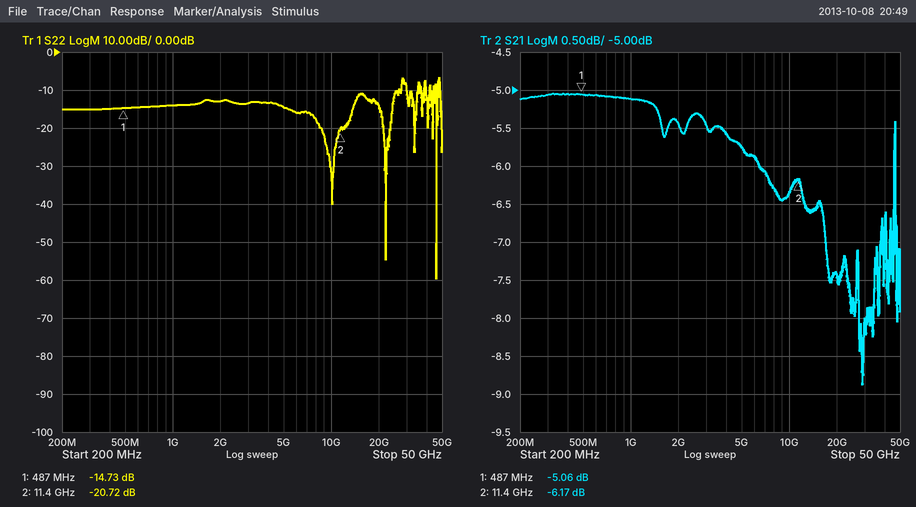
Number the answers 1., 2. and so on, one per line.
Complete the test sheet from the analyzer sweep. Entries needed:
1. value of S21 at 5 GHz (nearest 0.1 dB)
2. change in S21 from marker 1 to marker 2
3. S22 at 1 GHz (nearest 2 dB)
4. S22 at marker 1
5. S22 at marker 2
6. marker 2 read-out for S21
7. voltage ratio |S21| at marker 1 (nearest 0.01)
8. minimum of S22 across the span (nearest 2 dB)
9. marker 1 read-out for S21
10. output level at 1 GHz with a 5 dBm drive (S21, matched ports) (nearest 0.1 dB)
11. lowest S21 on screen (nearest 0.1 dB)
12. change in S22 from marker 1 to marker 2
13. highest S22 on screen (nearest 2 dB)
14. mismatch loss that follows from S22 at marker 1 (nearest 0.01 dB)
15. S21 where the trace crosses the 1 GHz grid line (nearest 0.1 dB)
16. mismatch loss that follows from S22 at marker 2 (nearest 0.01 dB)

1. -5.8 dB
2. -1.11 dB
3. -14 dB
4. -14.73 dB
5. -20.72 dB
6. -6.17 dB
7. 0.56
8. -60 dB
9. -5.06 dB
10. -0.1 dBm
11. -8.9 dB
12. -5.99 dB
13. -6 dB
14. 0.15 dB
15. -5.1 dB
16. 0.04 dB
